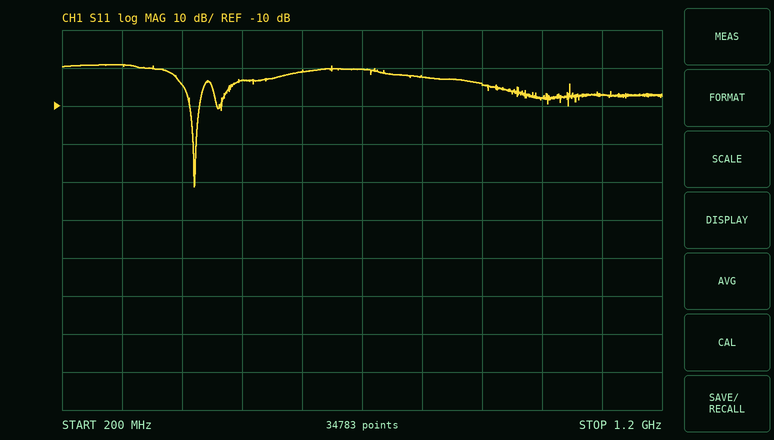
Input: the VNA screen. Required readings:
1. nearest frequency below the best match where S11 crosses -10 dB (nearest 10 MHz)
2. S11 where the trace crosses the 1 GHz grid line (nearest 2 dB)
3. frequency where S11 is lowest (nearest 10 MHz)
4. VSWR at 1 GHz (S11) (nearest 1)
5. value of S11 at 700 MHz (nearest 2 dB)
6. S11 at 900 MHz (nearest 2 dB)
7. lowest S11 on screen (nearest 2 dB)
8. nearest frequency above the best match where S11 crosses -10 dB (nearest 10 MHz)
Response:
410 MHz
-8 dB
420 MHz
2
0 dB
-4 dB
-32 dB
430 MHz
